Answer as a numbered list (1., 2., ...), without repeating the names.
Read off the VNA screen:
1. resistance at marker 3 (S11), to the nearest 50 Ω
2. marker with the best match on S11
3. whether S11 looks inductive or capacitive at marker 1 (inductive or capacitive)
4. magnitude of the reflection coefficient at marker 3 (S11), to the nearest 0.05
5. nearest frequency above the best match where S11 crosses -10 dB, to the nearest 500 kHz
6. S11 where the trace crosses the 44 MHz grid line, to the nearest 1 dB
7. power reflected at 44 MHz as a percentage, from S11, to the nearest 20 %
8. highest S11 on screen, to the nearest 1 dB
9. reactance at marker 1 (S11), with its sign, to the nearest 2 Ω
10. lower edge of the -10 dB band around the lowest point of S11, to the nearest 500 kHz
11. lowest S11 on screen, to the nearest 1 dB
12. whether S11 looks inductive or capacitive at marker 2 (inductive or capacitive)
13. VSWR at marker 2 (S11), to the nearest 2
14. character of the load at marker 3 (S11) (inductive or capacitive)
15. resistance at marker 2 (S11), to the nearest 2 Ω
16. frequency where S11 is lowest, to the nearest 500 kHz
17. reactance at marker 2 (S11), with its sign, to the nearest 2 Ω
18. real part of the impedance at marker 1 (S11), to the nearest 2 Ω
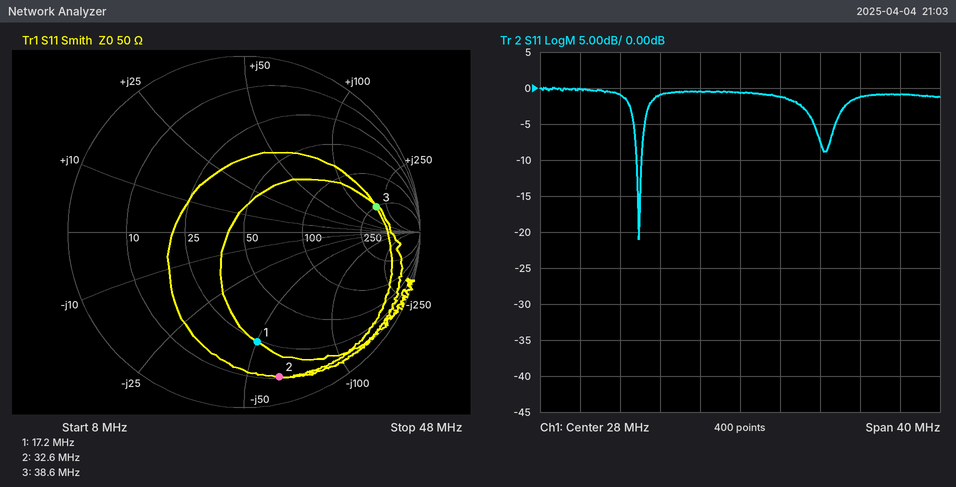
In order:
1. 250 Ω
2. marker 1
3. capacitive
4. 0.75
5. 18.0 MHz
6. -1 dB
7. 80 %
8. 0 dB
9. -50 Ω
10. 17.5 MHz
11. -21 dB
12. capacitive
13. 12
14. inductive
15. 10 Ω
16. 18.0 MHz
17. -62 Ω
18. 24 Ω
